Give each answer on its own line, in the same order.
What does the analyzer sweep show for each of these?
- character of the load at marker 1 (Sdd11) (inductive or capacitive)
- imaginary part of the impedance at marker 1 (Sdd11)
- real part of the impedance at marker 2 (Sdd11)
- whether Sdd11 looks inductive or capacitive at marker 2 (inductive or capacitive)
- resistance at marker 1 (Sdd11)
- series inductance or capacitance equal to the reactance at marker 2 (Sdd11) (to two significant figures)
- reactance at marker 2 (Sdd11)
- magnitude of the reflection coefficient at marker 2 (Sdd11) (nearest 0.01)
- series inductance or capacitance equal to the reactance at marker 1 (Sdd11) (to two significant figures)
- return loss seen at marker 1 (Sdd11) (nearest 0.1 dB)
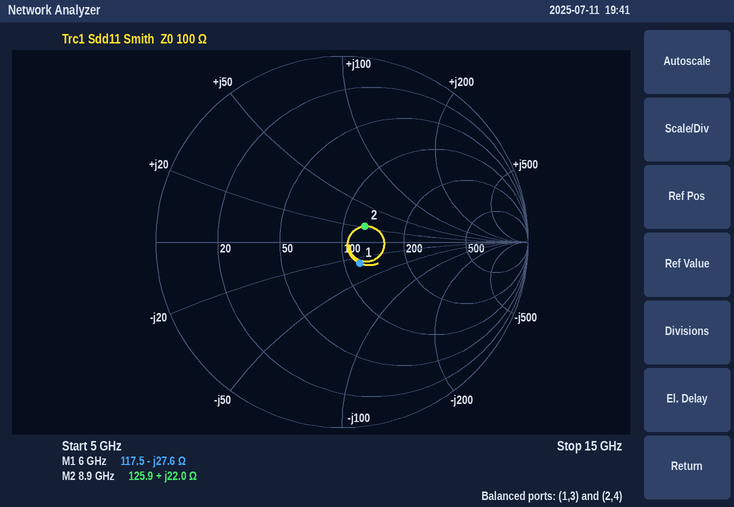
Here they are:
capacitive
-27.6 Ω
125.9 Ω
inductive
117.5 Ω
390 pH
+22.0 Ω
0.15
960 fF
16.5 dB
